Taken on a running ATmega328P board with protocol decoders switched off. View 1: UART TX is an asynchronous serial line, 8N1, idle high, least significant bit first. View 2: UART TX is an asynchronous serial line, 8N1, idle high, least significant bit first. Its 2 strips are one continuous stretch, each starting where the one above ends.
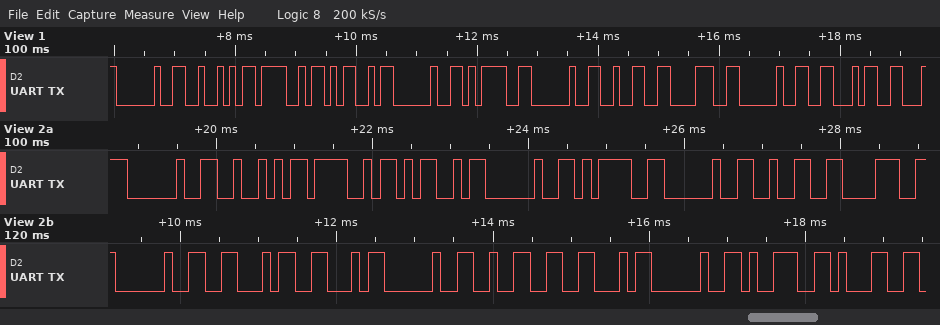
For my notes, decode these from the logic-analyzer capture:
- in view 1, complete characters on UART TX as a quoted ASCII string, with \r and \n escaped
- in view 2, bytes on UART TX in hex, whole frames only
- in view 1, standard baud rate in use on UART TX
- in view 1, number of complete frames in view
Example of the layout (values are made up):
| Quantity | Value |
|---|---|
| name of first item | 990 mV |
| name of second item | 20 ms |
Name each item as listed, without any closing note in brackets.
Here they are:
| Quantity | Value |
|---|---|
| in view 1, complete characters on UART TX as a quoted ASCII string, with \r and \n escaped | " ROM = 28 F" |
| in view 2, bytes on UART TX in hex, whole frames only | 20 52 4F 4D 20 3D 20 32 38 20 46 46 20 32 46 20 39 31 |
| in view 1, standard baud rate in use on UART TX | 9600 baud |
| in view 1, number of complete frames in view | 11 |
